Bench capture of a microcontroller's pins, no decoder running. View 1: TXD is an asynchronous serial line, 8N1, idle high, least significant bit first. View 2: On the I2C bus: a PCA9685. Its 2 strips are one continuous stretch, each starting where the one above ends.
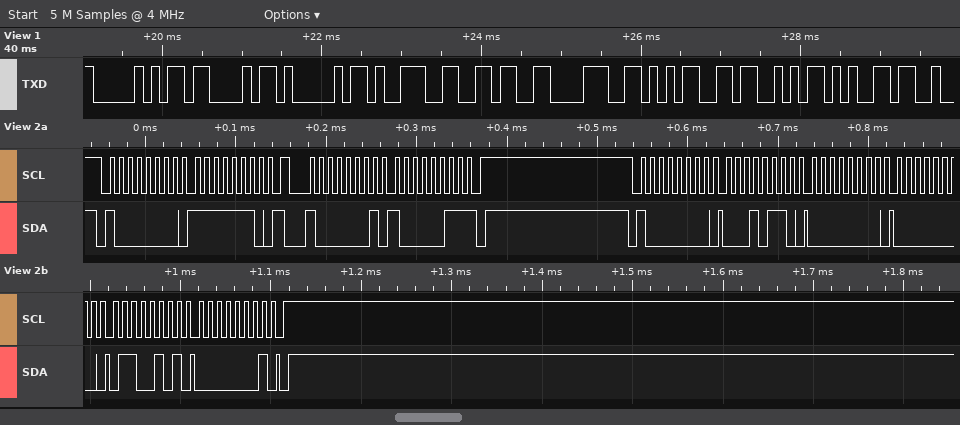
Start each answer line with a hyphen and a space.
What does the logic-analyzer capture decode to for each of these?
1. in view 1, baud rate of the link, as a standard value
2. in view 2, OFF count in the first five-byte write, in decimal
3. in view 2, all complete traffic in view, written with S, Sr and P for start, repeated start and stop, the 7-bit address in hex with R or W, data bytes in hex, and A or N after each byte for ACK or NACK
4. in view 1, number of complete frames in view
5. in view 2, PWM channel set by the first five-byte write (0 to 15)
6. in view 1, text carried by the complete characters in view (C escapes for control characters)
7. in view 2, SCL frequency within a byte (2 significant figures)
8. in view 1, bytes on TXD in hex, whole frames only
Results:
- 9600 baud
- 357
- S 40W A FE A Sr 40R A 83 N P S 40W A 16 A 00 A 00 A 65 A 01 A P
- 9
- 4
- "PCA9685Se"
- 100 kHz
- 0x50 0x43 0x41 0x39 0x36 0x38 0x35 0x53 0x65
